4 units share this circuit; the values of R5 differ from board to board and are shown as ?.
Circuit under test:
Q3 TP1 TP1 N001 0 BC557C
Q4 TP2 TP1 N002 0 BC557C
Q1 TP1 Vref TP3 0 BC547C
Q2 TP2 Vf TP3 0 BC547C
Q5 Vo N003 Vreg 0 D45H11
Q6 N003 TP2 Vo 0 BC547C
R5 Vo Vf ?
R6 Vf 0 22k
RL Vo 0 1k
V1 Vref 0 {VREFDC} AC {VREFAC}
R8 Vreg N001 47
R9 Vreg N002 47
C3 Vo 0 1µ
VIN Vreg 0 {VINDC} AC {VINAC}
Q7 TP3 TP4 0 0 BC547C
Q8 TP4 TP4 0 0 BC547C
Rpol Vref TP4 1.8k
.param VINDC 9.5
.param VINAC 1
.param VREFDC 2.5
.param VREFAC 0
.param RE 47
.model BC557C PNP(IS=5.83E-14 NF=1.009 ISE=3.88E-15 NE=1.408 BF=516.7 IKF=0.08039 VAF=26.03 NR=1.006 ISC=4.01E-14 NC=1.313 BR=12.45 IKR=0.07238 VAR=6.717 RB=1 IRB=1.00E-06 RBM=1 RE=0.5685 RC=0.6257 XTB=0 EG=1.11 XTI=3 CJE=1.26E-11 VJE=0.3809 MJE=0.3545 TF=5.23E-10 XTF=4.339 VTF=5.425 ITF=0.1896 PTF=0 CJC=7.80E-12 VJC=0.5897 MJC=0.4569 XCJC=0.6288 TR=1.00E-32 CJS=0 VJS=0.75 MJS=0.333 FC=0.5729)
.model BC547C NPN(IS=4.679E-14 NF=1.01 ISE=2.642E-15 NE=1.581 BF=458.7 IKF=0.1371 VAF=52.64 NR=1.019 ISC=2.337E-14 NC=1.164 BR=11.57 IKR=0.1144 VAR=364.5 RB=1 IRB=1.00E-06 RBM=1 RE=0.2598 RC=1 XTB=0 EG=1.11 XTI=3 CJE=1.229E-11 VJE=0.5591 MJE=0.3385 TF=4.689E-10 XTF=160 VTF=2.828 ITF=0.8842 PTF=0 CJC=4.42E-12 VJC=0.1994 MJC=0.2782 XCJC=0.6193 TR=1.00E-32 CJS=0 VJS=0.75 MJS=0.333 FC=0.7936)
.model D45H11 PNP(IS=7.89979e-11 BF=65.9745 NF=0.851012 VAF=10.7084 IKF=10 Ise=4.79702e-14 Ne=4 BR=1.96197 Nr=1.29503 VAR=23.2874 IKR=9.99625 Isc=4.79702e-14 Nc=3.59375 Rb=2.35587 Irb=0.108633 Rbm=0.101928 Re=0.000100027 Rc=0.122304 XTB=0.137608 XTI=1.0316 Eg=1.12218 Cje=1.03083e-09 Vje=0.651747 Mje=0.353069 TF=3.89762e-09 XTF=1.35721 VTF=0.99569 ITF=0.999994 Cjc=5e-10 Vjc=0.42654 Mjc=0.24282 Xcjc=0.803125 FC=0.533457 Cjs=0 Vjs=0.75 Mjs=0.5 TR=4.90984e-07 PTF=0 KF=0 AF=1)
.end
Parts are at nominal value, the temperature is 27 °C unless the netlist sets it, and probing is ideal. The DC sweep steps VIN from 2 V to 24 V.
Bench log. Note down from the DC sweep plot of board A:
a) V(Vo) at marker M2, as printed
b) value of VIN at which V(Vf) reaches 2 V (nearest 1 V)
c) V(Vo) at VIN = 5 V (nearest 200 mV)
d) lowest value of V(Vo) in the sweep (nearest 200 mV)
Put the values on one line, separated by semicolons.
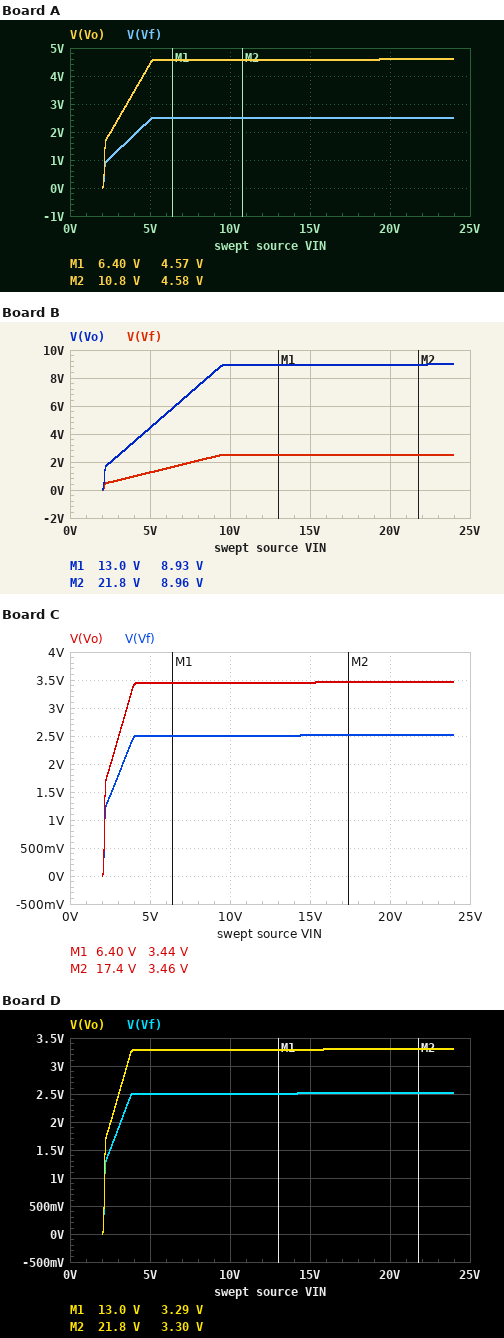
4.58 V; 4 V; 4.4 V; 0 V
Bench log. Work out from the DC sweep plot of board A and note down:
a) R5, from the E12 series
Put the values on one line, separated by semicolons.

18 kΩ
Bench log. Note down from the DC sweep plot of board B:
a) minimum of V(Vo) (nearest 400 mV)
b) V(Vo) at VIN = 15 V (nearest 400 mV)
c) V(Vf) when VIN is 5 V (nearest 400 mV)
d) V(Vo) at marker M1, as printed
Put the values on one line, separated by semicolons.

0 V; 8.8 V; 1.2 V; 8.93 V
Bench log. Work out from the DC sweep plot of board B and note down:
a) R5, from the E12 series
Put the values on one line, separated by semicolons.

56 kΩ
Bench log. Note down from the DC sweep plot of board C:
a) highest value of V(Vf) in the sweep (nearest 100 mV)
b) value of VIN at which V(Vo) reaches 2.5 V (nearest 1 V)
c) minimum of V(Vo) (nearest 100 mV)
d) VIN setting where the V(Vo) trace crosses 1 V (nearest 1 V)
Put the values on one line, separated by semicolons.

2.5 V; 3 V; 0 V; 2 V
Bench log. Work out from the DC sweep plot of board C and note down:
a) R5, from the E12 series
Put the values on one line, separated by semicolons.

8.2 kΩ
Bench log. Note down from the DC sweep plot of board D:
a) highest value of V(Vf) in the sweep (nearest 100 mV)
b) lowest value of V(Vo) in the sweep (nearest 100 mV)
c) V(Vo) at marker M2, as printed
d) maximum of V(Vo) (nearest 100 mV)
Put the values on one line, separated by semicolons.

2.5 V; 0 V; 3.30 V; 3.3 V
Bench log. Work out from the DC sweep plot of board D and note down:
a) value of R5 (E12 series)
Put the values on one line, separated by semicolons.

6.8 kΩ
